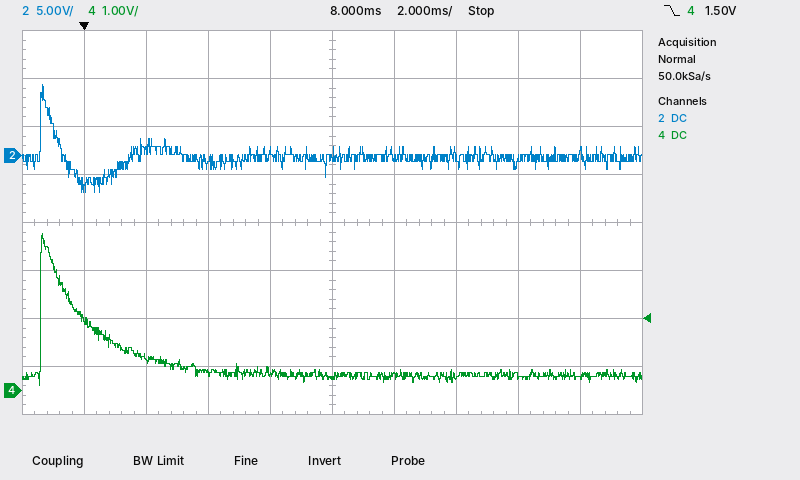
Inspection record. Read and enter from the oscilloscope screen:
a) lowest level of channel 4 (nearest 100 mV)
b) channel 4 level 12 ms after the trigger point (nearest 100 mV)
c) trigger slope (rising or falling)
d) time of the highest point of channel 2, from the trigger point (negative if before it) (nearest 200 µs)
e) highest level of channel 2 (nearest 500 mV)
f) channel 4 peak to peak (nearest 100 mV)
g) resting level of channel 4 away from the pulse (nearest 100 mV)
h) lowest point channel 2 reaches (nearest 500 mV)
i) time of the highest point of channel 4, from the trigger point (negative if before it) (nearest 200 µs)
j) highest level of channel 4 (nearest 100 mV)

100 mV
300 mV
falling
-1.4 ms
7.5 V
3.2 V
300 mV
-4.0 V
-1.4 ms
3.3 V
